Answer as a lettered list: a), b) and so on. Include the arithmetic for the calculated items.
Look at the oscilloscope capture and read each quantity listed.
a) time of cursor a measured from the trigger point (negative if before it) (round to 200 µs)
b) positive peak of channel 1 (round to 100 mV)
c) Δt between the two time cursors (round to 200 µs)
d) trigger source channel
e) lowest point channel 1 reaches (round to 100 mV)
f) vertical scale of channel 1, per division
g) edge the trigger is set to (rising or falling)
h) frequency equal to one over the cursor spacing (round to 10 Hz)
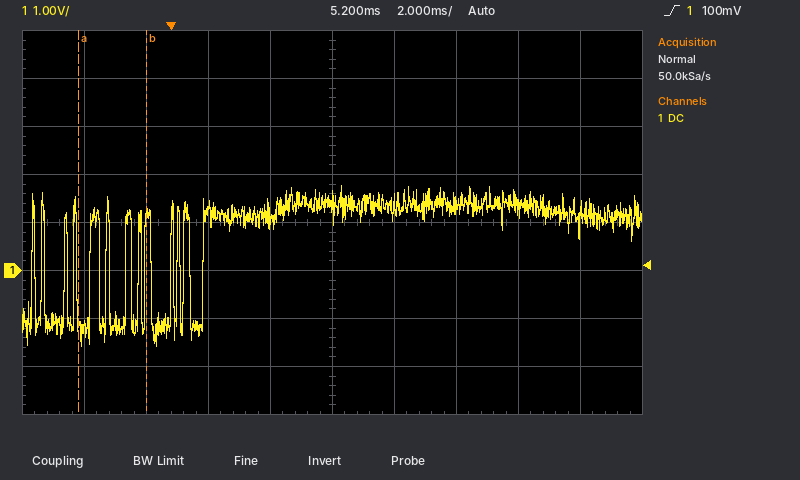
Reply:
a) -3.0 ms
b) 1.8 V
c) 2.2 ms
d) channel 1
e) -1.6 V
f) 1 V
g) rising
h) 1 / 2.2 ms ≈ 450 Hz
